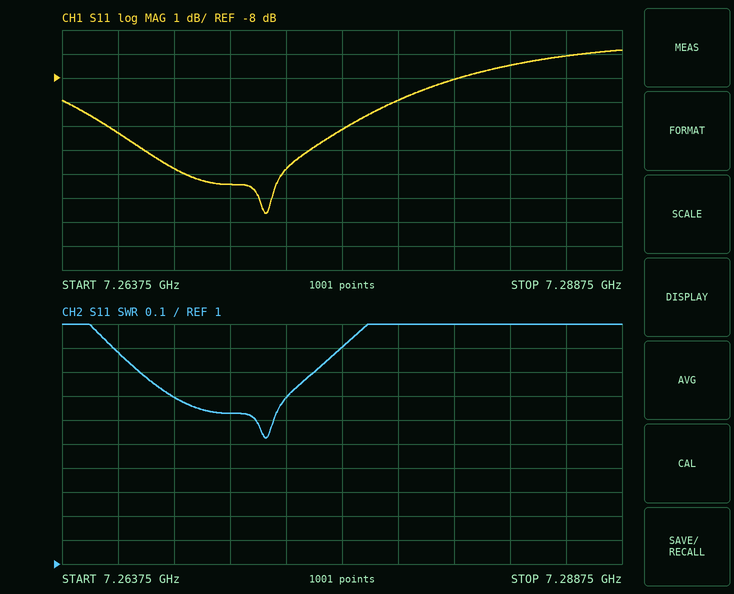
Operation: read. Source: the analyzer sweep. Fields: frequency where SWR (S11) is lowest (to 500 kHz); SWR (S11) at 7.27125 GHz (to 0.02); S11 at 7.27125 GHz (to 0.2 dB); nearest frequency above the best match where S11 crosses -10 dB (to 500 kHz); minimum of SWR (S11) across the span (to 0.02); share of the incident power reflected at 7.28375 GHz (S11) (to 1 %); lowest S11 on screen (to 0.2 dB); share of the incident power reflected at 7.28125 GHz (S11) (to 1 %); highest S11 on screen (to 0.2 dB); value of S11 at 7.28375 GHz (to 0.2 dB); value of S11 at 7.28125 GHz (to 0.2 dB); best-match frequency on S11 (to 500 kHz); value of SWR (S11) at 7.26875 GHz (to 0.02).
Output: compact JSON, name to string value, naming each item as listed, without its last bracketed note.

{"frequency where SWR (S11) is lowest": "7.2730 GHz", "SWR (S11) at 7.27125 GHz": "1.62", "S11 at 7.27125 GHz": "-12.4 dB", "nearest frequency above the best match where S11 crosses -10 dB": "7.2765 GHz", "minimum of SWR (S11) across the span": "1.52", "share of the incident power reflected at 7.28375 GHz (S11)": "18 %", "lowest S11 on screen": "-13.6 dB", "share of the incident power reflected at 7.28125 GHz (S11)": "16 %", "highest S11 on screen": "-6.8 dB", "value of S11 at 7.28375 GHz": "-7.4 dB", "value of S11 at 7.28125 GHz": "-8.0 dB", "best-match frequency on S11": "7.2730 GHz", "value of SWR (S11) at 7.26875 GHz": "1.70"}
